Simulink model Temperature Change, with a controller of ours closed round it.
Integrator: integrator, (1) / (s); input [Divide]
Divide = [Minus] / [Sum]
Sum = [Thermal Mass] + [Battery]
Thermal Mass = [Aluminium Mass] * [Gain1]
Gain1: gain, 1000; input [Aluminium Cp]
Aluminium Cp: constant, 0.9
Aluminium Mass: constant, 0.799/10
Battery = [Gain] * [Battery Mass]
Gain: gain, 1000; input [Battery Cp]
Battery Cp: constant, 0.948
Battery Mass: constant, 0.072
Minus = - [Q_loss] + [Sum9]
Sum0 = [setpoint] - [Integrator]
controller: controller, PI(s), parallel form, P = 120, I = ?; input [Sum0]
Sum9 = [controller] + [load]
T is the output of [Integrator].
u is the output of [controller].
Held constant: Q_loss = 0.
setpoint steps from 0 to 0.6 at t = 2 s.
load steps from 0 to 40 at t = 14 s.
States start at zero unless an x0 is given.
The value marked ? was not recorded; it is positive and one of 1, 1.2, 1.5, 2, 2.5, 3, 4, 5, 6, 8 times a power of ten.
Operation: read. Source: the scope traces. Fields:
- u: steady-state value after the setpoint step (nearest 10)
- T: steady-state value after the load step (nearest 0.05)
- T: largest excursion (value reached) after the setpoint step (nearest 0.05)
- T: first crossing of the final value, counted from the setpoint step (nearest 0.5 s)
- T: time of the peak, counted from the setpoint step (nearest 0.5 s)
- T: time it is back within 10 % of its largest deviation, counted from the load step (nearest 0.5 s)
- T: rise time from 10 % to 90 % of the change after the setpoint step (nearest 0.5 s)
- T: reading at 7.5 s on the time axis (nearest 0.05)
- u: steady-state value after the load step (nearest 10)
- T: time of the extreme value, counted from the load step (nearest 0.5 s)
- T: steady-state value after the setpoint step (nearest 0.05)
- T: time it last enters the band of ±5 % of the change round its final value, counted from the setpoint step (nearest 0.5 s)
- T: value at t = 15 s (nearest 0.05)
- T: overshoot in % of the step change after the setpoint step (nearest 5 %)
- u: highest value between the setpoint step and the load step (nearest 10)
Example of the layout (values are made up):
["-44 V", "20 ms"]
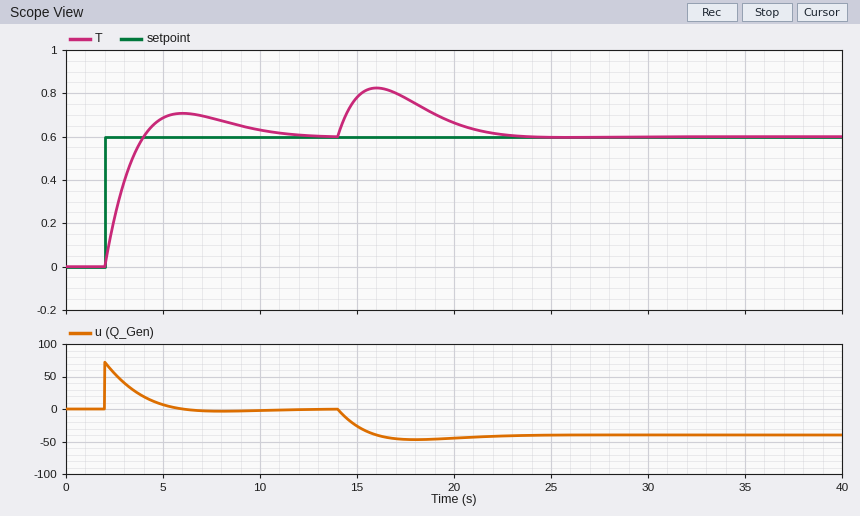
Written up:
["0", "0.60", "0.70", "2.0 s", "4.0 s", "7.5 s", "1.5 s", "0.70", "-40", "2.0 s", "0.60", "8.0 s", "0.80", "20 %", "70"]
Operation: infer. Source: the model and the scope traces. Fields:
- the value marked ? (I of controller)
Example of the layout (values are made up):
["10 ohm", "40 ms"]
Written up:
["40"]
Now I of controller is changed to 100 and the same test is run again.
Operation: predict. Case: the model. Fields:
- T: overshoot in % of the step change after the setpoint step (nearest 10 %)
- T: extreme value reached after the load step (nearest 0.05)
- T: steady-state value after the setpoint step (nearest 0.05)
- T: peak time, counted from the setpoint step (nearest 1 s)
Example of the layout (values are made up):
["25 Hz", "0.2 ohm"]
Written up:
["30 %", "0.80", "0.60", "3 s"]
